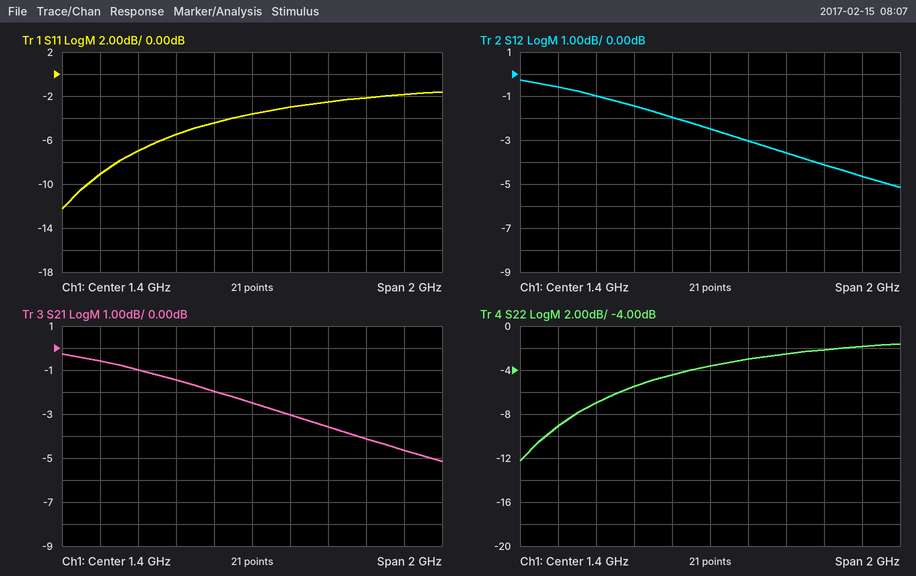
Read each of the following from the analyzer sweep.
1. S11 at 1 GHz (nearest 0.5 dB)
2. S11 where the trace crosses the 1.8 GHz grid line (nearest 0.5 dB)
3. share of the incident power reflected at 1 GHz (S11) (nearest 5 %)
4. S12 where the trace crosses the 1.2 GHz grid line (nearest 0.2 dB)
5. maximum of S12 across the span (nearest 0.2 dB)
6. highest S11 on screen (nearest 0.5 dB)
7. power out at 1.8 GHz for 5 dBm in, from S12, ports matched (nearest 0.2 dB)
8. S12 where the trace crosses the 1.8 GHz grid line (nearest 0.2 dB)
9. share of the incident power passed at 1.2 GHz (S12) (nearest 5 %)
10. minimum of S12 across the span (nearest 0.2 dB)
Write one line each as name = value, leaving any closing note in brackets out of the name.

S11 at 1 GHz = -5.5 dB
S11 where the trace crosses the 1.8 GHz grid line = -2.5 dB
share of the incident power reflected at 1 GHz (S11) = 30 %
S12 where the trace crosses the 1.2 GHz grid line = -2.0 dB
maximum of S12 across the span = -0.2 dB
highest S11 on screen = -1.5 dB
power out at 1.8 GHz for 5 dBm in, from S12, ports matched = 1.4 dBm
S12 where the trace crosses the 1.8 GHz grid line = -3.6 dB
share of the incident power passed at 1.2 GHz (S12) = 65 %
minimum of S12 across the span = -5.2 dB
